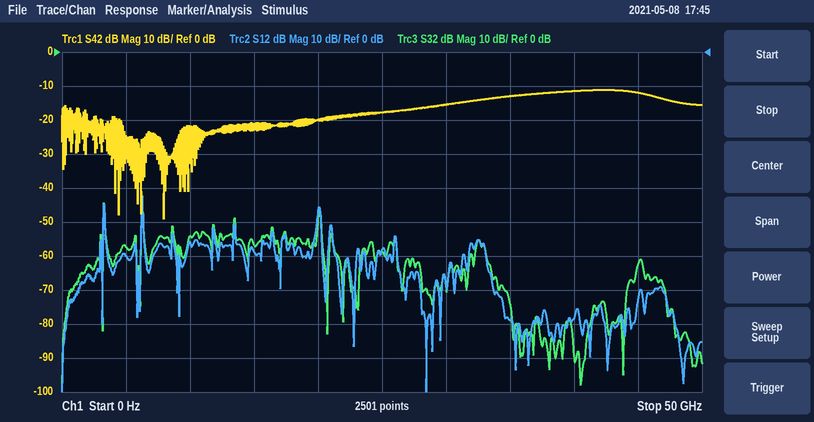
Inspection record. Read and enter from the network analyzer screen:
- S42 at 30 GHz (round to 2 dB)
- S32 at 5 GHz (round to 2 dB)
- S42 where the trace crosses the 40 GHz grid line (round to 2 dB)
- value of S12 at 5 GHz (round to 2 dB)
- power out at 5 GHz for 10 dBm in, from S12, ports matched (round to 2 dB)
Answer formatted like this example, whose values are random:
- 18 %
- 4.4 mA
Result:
- -16 dB
- -58 dB
- -12 dB
- -60 dB
- -50 dBm
